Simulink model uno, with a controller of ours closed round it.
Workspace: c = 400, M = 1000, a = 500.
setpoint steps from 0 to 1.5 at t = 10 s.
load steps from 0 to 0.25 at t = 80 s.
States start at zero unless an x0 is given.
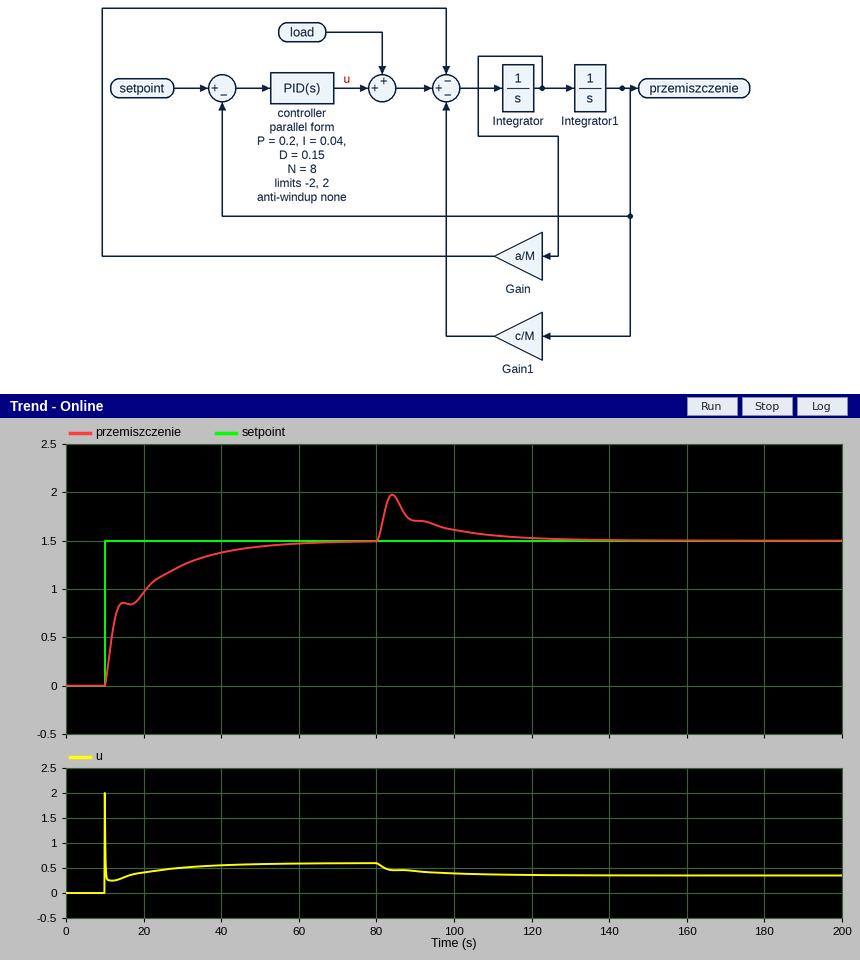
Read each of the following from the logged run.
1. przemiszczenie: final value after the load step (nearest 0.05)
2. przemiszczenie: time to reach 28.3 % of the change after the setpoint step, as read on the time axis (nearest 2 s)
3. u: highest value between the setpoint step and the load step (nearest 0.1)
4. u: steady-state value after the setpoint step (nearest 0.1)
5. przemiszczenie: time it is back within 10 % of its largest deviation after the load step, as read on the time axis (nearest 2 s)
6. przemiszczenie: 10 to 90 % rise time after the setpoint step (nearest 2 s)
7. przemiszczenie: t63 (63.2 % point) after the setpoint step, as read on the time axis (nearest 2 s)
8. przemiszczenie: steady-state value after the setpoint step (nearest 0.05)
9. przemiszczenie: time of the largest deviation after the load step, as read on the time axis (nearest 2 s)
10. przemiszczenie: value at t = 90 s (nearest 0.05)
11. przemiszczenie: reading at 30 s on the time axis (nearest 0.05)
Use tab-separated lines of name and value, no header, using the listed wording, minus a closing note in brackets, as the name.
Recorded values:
przemiszczenie: final value after the load step	1.50
przemiszczenie: time to reach 28.3 % of the change after the setpoint step, as read on the time axis	12 s
u: highest value between the setpoint step and the load step	2.0
u: steady-state value after the setpoint step	0.6
przemiszczenie: time it is back within 10 % of its largest deviation after the load step, as read on the time axis	112 s
przemiszczenie: 10 to 90 % rise time after the setpoint step	26 s
przemiszczenie: t63 (63.2 % point) after the setpoint step, as read on the time axis	20 s
przemiszczenie: steady-state value after the setpoint step	1.50
przemiszczenie: time of the largest deviation after the load step, as read on the time axis	84 s
przemiszczenie: value at t = 90 s	1.70
przemiszczenie: reading at 30 s on the time axis	1.25
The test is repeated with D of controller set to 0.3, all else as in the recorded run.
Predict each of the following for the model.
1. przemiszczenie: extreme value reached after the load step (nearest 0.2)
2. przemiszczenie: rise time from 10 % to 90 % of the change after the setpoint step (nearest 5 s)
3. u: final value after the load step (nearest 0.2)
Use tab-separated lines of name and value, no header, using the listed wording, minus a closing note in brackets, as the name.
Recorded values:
przemiszczenie: extreme value reached after the load step	2.0
przemiszczenie: rise time from 10 % to 90 % of the change after the setpoint step	25 s
u: final value after the load step	0.4
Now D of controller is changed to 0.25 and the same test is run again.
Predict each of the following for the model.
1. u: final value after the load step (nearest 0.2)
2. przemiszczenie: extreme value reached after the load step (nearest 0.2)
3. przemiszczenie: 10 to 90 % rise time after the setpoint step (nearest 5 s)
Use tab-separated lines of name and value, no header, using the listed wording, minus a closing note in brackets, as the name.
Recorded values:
u: final value after the load step	0.4
przemiszczenie: extreme value reached after the load step	2.0
przemiszczenie: 10 to 90 % rise time after the setpoint step	25 s
